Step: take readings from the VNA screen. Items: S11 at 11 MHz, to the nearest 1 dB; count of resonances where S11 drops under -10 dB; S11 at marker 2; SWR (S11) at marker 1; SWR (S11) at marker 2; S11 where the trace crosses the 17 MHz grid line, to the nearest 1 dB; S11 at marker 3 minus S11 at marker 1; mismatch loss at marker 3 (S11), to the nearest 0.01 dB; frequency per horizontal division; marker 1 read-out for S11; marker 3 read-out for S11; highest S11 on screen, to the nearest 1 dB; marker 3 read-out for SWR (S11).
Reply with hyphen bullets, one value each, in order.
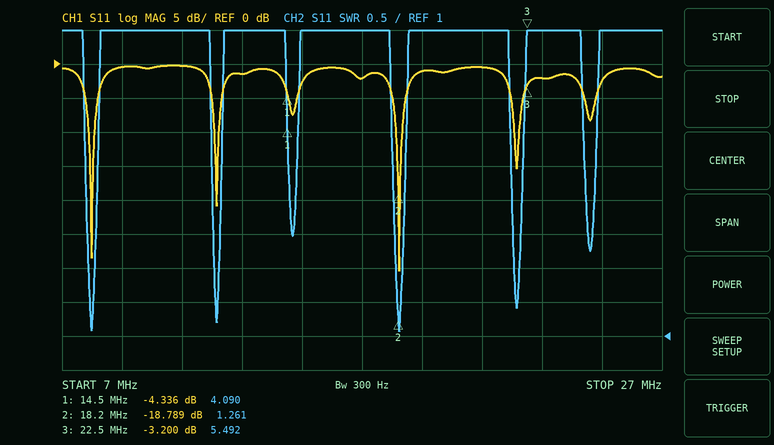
- 0 dB
- 4
- -18.789 dB
- 4.090
- 1.261
- -2 dB
- 1.136 dB
- 2.83 dB
- 2 MHz
- -4.336 dB
- -3.200 dB
- 0 dB
- 5.492
